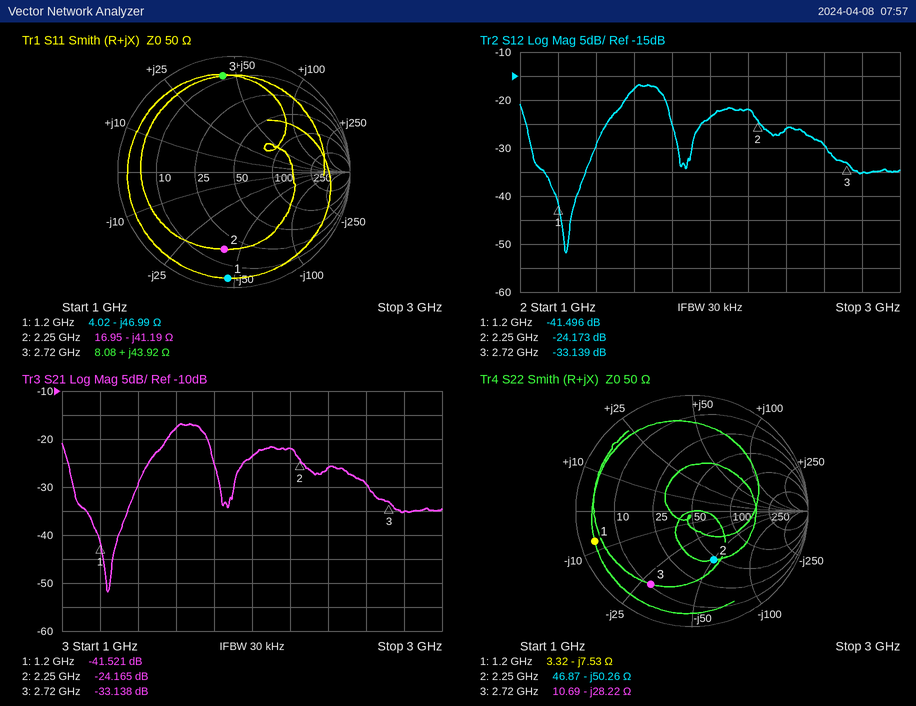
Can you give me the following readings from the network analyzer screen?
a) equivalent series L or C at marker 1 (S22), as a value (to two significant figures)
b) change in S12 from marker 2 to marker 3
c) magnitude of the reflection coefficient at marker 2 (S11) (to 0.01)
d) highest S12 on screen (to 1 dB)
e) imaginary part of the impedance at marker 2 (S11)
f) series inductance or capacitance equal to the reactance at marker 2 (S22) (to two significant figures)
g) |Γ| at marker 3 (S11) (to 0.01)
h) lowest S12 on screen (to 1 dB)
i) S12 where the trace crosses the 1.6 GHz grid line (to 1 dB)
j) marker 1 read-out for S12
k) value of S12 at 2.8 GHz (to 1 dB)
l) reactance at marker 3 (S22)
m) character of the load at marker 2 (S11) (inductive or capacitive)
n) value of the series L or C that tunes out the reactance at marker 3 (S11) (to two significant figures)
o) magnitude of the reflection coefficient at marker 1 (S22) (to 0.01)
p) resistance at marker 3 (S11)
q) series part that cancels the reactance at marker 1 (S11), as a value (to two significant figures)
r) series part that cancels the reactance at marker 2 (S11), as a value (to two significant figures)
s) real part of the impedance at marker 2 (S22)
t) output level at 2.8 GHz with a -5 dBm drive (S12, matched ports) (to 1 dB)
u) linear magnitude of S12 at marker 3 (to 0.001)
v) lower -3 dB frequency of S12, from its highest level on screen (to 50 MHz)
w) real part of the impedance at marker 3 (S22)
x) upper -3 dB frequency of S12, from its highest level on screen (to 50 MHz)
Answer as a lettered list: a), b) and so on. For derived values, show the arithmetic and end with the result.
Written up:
a) C = 1/(2π × 1.2 GHz × 7.53 Ω) ≈ 18 pF
b) -33.139 − (-24.173) = -8.966 dB
c) 0.67
d) -17 dB
e) -41.19 Ω
f) C = 1/(2π × 2.25 GHz × 50.26 Ω) ≈ 1.4 pF
g) 0.83
h) -52 dB
i) -18 dB
j) -41.496 dB
k) -35 dB
l) -28.22 Ω
m) capacitive
n) C = 1/(2π × 2.72 GHz × 43.92 Ω) ≈ 1.3 pF
o) 0.88
p) 8.08 Ω
q) L = 46.99 Ω/(2π × 1.2 GHz) ≈ 6.2 nH
r) L = 41.19 Ω/(2π × 2.25 GHz) ≈ 2.9 nH
s) 46.87 Ω
t) -5 dBm + (-35 dB) = -40 dBm
u) 10^(-33.139/20) ≈ 0.022
v) 1.55 GHz
w) 10.69 Ω
x) 1.75 GHz
